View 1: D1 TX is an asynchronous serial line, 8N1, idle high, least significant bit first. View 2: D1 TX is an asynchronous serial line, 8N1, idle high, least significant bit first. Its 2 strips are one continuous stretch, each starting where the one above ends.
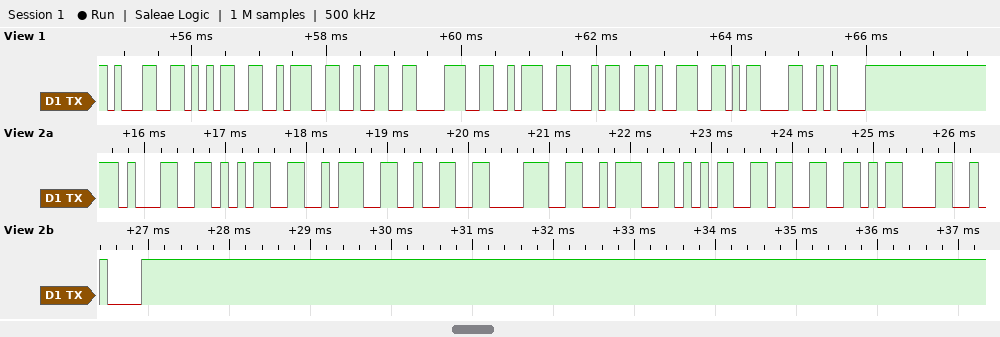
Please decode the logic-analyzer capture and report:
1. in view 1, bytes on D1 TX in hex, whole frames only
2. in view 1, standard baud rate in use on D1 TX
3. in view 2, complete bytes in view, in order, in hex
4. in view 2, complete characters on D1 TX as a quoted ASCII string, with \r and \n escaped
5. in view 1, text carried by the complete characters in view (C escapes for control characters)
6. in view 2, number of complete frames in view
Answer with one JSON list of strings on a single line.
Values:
["31 35 3A 32 38 3A 34 39 0D 0A", "9600 baud", "31 35 3A 32 38 3A 35 33 0D 0A", "\"15:28:53\\r\\n\"", "\"15:28:49\\r\\n\"", "10"]
